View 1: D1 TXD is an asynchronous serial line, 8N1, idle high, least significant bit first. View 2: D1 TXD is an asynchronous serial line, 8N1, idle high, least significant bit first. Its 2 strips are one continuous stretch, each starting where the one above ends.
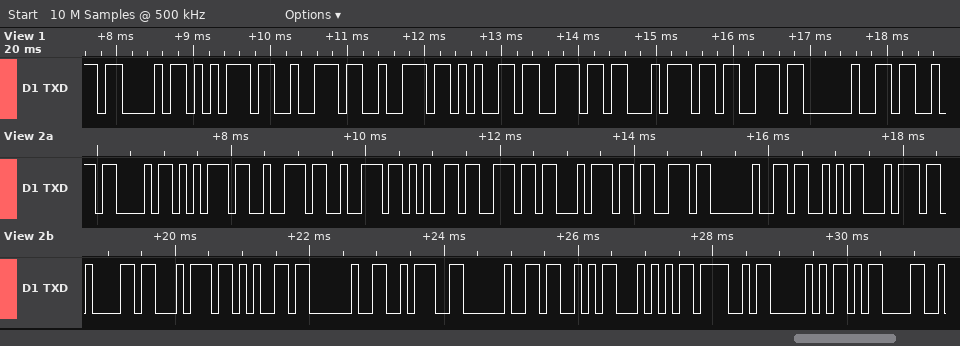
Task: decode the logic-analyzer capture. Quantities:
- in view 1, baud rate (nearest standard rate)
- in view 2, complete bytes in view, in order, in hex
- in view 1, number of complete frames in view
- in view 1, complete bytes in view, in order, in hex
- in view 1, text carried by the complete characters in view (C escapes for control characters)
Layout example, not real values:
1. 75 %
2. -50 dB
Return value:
1. 9600 baud
2. 0x43 0x75 0x72 0x72 0x65 0x6E 0x74 0x73 0x20 0x53 0x74 0x61 0x74 0x65 0x20 0x3A 0x20 0x53 0x54 0x4F 0x50 0x0D
3. 9
4. 43 75 72 72 65 6E 74 73 20
5. "Currents "
